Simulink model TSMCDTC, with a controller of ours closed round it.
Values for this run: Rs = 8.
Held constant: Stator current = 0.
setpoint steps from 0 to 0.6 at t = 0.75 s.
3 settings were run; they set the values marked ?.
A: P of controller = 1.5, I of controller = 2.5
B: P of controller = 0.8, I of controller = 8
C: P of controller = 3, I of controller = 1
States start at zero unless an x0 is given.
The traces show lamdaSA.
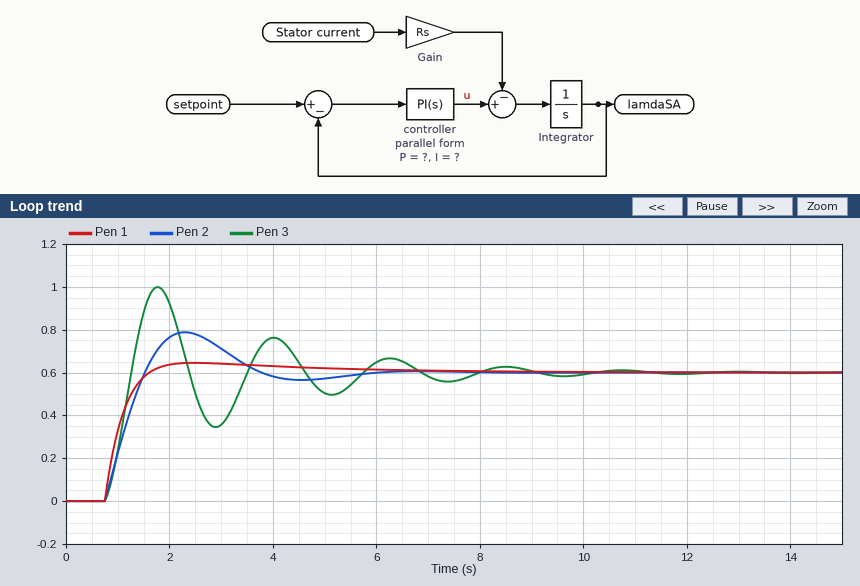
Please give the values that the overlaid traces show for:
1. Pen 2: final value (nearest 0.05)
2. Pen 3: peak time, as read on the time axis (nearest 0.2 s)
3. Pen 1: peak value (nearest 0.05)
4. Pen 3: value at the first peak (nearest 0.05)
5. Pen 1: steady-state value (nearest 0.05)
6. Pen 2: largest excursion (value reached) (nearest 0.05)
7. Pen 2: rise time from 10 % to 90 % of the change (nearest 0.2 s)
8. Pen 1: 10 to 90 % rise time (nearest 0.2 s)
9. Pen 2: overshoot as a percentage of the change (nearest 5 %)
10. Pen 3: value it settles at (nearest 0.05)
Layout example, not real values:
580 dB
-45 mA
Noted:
0.60
1.8 s
0.65
1.00
0.60
0.80
0.6 s
0.6 s
30 %
0.60
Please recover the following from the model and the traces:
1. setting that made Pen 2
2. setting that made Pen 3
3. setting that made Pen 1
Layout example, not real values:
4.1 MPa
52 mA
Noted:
A
B
C
